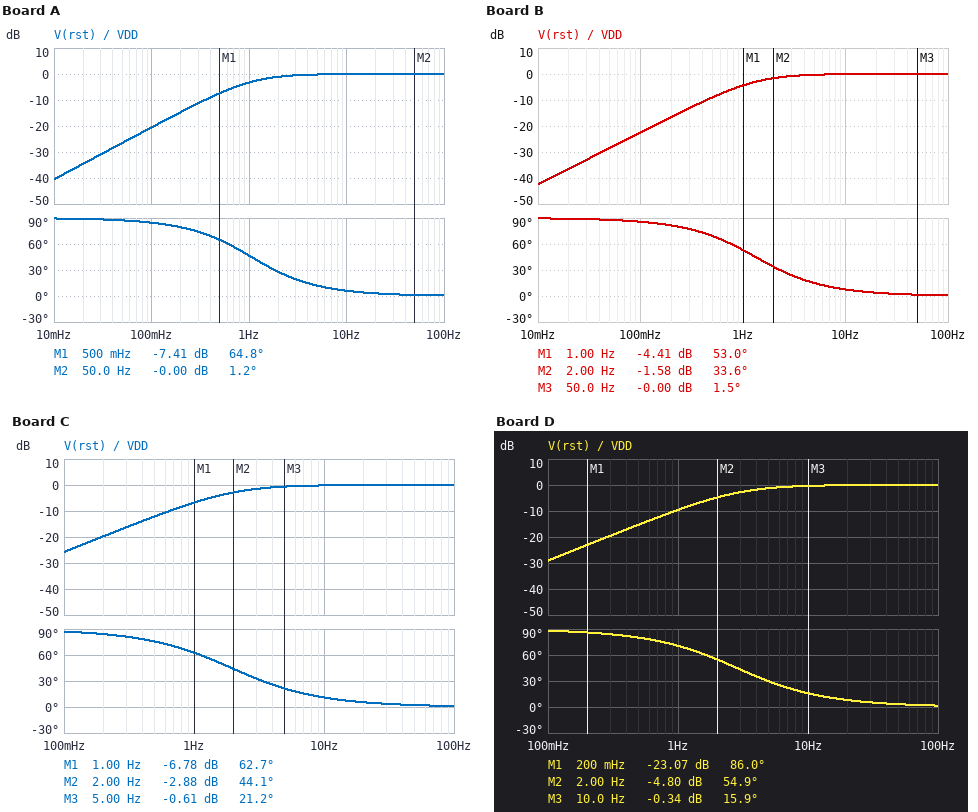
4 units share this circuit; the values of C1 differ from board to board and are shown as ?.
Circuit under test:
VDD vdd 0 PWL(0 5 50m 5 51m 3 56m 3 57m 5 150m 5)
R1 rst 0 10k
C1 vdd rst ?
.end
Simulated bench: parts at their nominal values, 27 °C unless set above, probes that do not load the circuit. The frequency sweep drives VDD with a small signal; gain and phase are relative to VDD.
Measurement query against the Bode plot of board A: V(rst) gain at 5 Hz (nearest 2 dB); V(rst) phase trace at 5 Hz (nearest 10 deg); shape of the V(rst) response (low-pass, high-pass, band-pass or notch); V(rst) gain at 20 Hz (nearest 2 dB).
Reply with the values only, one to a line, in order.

0 dB
10 deg
high-pass
0 dB
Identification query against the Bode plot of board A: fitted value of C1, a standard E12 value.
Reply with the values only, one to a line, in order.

15 µF
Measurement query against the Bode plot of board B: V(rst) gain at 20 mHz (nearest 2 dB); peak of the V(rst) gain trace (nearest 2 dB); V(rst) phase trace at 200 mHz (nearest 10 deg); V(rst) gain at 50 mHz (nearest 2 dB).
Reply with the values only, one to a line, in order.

-36 dB
0 dB
80 deg
-28 dB
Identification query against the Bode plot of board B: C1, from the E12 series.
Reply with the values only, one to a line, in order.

12 µF
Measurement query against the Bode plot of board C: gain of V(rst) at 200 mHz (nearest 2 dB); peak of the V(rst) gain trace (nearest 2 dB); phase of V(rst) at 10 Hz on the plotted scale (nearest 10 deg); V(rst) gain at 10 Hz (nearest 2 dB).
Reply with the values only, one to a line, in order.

-20 dB
0 dB
10 deg
0 dB
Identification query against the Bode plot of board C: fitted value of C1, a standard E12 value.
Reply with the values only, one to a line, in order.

8.2 µF
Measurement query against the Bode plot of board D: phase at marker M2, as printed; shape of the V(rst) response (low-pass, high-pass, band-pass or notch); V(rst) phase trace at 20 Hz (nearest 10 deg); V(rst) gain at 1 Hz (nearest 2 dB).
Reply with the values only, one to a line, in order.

54.9 deg
high-pass
10 deg
-10 dB
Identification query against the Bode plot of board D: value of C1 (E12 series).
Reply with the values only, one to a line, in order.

5.6 µF
